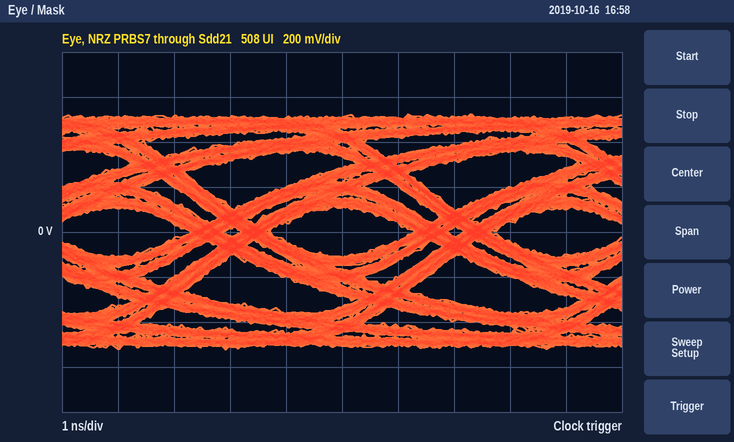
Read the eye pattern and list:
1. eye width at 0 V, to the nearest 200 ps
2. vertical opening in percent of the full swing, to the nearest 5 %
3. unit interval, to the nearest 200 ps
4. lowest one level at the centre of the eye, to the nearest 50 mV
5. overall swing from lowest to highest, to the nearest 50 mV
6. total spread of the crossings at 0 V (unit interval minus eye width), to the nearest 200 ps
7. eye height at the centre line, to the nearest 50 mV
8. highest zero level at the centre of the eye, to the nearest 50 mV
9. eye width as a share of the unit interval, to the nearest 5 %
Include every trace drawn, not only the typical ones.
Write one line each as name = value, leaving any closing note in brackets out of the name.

eye width at 0 V, to the nearest 200 ps = 2.6 ns
vertical opening in percent of the full swing, to the nearest 5 % = 20 %
unit interval, to the nearest 200 ps = 4.0 ns
lowest one level at the centre of the eye, to the nearest 50 mV = 100 mV
overall swing from lowest to highest, to the nearest 50 mV = 1.05 V
total spread of the crossings at 0 V (unit interval minus eye width), to the nearest 200 ps = 1.4 ns
eye height at the centre line, to the nearest 50 mV = 200 mV
highest zero level at the centre of the eye, to the nearest 50 mV = -100 mV
eye width as a share of the unit interval, to the nearest 5 % = 65 %
